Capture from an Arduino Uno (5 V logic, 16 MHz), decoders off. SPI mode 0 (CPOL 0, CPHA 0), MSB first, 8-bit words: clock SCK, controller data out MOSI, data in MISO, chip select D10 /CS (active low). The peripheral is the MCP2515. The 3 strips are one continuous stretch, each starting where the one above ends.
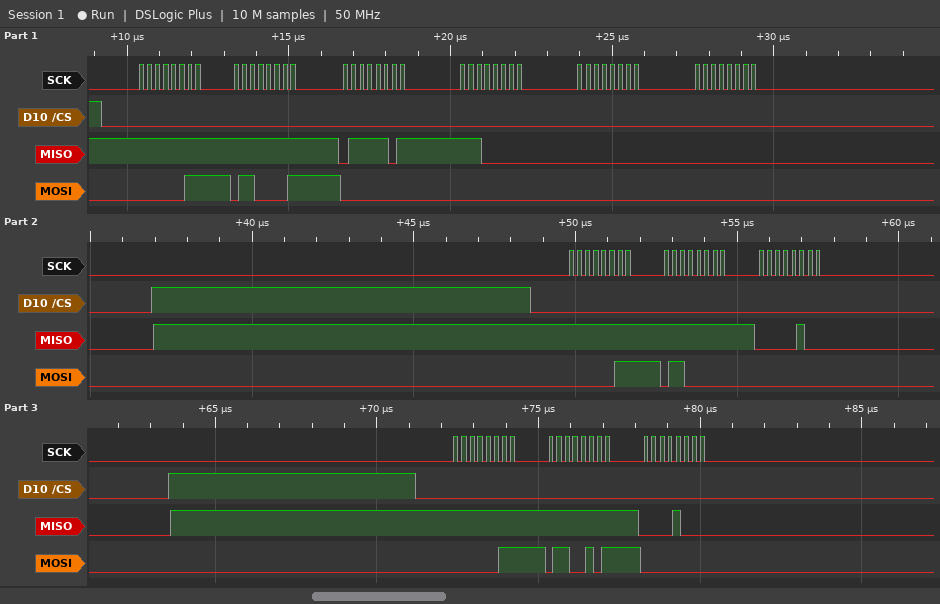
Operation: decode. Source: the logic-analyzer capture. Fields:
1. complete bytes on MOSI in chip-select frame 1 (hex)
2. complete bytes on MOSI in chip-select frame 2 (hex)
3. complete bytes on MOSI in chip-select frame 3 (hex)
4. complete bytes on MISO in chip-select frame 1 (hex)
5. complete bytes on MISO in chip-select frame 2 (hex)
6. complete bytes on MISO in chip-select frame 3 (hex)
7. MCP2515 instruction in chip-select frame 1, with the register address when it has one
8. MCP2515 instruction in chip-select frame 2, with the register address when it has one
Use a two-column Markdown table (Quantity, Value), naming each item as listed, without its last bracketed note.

| Quantity | Value |
|---|---|
| complete bytes on MOSI in chip-select frame 1 | 0x03 0x61 0x00 0x00 0x00 0x00 |
| complete bytes on MOSI in chip-select frame 2 | 0x03 0x60 0x00 |
| complete bytes on MOSI in chip-select frame 3 | 0x03 0x65 0x00 |
| complete bytes on MISO in chip-select frame 1 | 0xFF 0xFF 0x7D 0xE0 0x00 0x00 |
| complete bytes on MISO in chip-select frame 2 | 0xFF 0xFF 0x04 |
| complete bytes on MISO in chip-select frame 3 | 0xFF 0xFF 0x08 |
| MCP2515 instruction in chip-select frame 1, with the register address when it has one | READ 0x61 |
| MCP2515 instruction in chip-select frame 2, with the register address when it has one | READ 0x60 |
